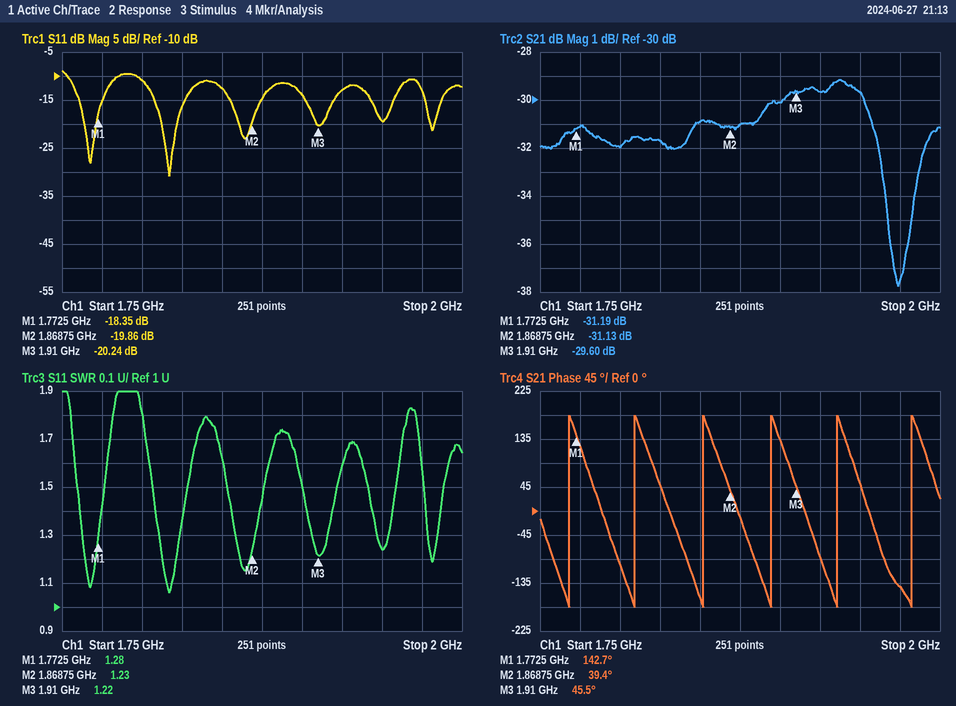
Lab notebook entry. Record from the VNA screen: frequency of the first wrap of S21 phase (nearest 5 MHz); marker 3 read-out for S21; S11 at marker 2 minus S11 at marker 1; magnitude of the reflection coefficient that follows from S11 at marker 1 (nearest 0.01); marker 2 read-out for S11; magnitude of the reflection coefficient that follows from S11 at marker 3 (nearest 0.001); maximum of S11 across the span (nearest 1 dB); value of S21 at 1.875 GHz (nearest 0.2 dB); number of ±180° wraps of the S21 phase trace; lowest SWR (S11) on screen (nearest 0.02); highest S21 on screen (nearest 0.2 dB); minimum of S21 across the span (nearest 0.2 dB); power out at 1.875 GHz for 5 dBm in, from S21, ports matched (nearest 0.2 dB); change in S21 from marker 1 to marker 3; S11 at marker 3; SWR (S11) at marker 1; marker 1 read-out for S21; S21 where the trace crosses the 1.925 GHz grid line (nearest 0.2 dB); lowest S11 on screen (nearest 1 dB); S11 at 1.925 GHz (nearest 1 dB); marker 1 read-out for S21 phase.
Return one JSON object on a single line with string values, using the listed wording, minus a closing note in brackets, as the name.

{"frequency of the first wrap of S21 phase": "1.770 GHz", "marker 3 read-out for S21": "-29.60 dB", "S11 at marker 2 minus S11 at marker 1": "-1.51 dB", "magnitude of the reflection coefficient that follows from S11 at marker 1": "0.12", "marker 2 read-out for S11": "-19.86 dB", "magnitude of the reflection coefficient that follows from S11 at marker 3": "0.097", "maximum of S11 across the span": "-9 dB", "value of S21 at 1.875 GHz": "-31.0 dB", "number of ±180° wraps of the S21 phase trace": "6", "lowest SWR (S11) on screen": "1.06", "highest S21 on screen": "-29.2 dB", "minimum of S21 across the span": "-37.8 dB", "power out at 1.875 GHz for 5 dBm in, from S21, ports matched": "-26.0 dBm", "change in S21 from marker 1 to marker 3": "1.59 dB", "S11 at marker 3": "-20.24 dB", "SWR (S11) at marker 1": "1.28", "marker 1 read-out for S21": "-31.19 dB", "S21 where the trace crosses the 1.925 GHz grid line": "-29.6 dB", "lowest S11 on screen": "-31 dB", "S11 at 1.925 GHz": "-13 dB", "marker 1 read-out for S21 phase": "142.7°"}
